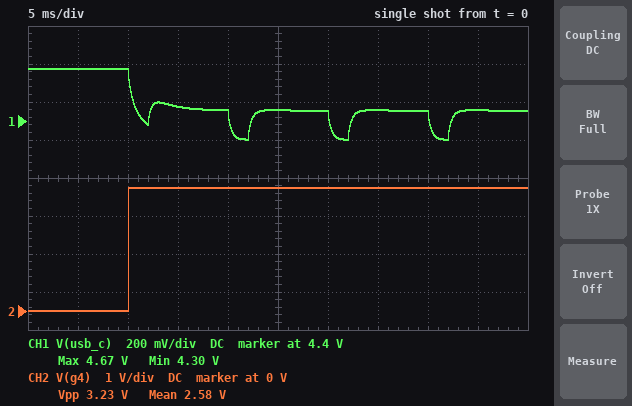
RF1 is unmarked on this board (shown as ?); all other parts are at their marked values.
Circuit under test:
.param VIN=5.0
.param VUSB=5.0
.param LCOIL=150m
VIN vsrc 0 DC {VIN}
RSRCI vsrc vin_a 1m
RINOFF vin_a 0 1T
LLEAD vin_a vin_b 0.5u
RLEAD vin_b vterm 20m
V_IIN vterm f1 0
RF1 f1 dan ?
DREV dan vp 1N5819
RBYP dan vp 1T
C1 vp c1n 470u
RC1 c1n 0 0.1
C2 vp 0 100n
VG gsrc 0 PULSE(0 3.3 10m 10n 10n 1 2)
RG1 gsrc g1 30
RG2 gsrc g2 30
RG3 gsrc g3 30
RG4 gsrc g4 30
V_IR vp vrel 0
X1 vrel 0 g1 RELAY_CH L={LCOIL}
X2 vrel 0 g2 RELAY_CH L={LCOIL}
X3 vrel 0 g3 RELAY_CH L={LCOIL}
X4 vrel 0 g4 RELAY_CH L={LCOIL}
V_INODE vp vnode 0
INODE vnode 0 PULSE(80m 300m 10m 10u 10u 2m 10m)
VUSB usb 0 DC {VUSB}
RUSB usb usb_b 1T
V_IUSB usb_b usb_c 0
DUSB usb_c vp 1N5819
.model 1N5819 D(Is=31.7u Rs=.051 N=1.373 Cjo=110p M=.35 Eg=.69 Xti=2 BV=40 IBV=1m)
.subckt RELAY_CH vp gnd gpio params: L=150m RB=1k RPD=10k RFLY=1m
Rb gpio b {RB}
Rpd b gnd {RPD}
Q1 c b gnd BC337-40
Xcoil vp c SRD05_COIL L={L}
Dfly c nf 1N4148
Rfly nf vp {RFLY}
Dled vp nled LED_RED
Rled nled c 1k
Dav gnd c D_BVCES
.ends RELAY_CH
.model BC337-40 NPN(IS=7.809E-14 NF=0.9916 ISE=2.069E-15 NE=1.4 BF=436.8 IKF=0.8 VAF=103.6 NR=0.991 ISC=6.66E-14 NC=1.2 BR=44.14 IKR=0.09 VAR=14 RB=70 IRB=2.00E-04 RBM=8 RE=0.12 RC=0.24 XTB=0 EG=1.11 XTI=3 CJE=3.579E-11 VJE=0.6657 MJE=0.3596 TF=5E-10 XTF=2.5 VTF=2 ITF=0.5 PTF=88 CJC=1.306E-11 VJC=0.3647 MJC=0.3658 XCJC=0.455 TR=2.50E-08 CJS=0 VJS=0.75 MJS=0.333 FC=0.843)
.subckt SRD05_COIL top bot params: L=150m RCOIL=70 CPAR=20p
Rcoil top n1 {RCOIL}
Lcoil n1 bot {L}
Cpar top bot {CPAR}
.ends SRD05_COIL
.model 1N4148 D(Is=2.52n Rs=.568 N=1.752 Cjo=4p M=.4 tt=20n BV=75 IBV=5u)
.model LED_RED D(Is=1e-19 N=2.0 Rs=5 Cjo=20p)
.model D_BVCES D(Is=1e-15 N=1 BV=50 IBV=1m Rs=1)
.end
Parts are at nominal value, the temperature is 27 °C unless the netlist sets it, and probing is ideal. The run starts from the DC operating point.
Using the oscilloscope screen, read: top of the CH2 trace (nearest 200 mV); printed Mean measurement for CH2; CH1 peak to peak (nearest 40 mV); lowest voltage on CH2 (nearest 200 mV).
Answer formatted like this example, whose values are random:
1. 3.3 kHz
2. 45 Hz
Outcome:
1. 3.2 V
2. 2.58 V
3. 360 mV
4. 0 V
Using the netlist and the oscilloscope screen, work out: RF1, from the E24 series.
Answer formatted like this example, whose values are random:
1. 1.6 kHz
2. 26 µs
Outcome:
1. 0.56 Ω
